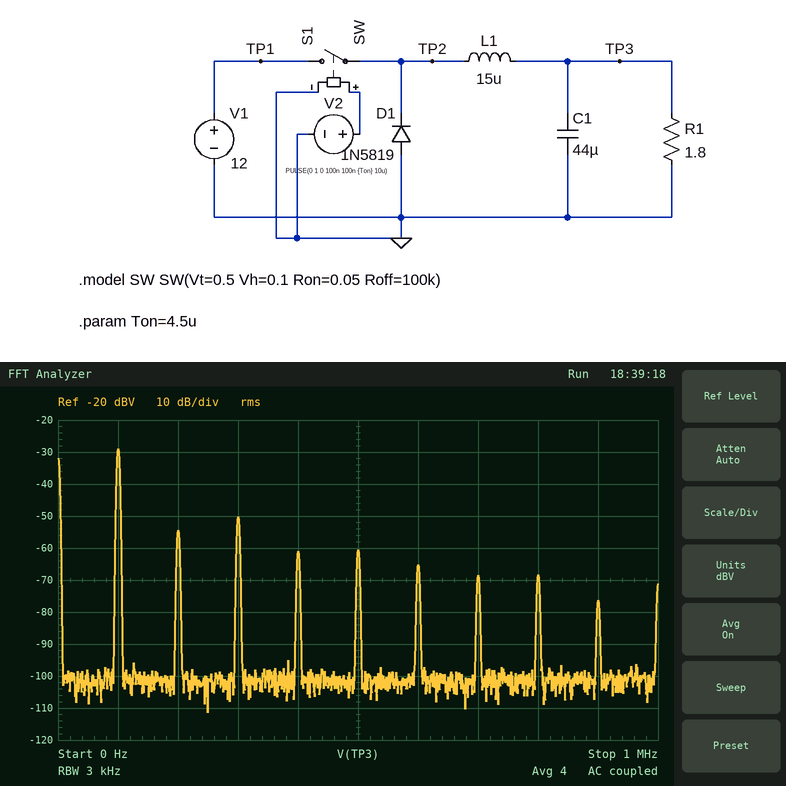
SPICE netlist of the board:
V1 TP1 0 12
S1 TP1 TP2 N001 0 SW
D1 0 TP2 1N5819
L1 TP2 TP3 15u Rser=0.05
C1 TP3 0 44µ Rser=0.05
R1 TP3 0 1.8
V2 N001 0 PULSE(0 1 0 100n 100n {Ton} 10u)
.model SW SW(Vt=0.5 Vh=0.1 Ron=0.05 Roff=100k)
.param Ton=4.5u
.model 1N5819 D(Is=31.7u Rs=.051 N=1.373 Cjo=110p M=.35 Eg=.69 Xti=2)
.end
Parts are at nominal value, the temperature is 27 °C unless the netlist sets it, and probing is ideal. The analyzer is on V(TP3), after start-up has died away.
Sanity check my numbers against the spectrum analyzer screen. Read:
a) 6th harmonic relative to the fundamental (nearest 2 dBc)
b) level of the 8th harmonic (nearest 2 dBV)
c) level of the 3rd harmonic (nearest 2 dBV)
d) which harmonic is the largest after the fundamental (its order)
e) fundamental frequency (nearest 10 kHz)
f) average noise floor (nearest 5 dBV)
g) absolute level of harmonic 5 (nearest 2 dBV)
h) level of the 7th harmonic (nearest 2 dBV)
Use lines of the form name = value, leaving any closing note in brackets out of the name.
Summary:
6th harmonic relative to the fundamental = -36 dBc
level of the 8th harmonic = -68 dBV
level of the 3rd harmonic = -50 dBV
which harmonic is the largest after the fundamental = 3
fundamental frequency = 100 kHz
average noise floor = -100 dBV
absolute level of harmonic 5 = -60 dBV
level of the 7th harmonic = -68 dBV
